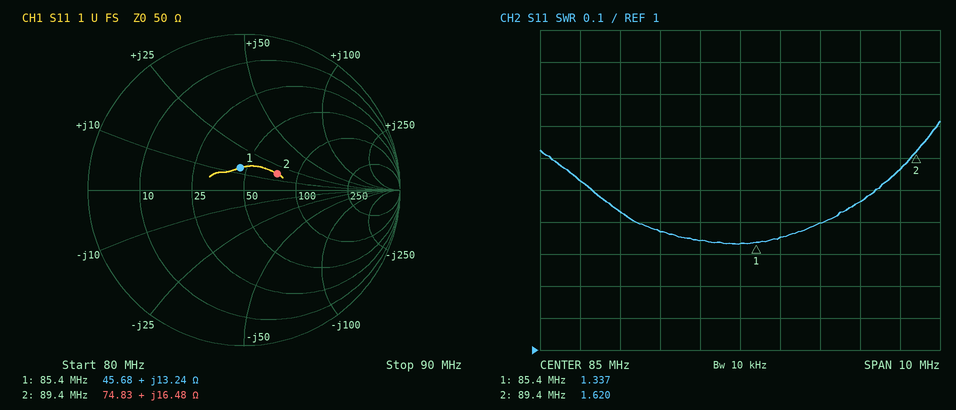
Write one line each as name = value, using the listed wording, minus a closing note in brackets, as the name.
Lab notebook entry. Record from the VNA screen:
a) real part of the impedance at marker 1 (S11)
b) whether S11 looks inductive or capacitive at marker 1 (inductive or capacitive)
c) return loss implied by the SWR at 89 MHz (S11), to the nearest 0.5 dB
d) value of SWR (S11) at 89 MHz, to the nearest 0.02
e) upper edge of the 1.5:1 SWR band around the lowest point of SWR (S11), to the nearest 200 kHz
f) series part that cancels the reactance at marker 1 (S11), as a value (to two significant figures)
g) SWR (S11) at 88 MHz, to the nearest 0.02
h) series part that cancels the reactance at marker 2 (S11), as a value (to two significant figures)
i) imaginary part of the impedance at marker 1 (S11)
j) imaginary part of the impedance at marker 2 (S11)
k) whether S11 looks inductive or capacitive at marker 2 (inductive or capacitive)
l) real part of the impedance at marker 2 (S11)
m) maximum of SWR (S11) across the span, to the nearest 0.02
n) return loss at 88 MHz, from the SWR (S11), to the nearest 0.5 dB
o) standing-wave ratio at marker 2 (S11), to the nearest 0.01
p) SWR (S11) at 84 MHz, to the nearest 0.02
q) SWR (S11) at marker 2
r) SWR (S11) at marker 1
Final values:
real part of the impedance at marker 1 = 45.68 Ω
whether S11 looks inductive or capacitive at marker 1 = inductive
return loss implied by the SWR at 89 MHz (S11), to the nearest 0.5 dB = 13.0 dB
value of SWR (S11) at 89 MHz, to the nearest 0.02 = 1.56
upper edge of the 1.5:1 SWR band around the lowest point of SWR (S11), to the nearest 200 kHz = 88.4 MHz
series part that cancels the reactance at marker 1 (S11), as a value = 140 pF
SWR (S11) at 88 MHz, to the nearest 0.02 = 1.46
series part that cancels the reactance at marker 2 (S11), as a value = 110 pF
imaginary part of the impedance at marker 1 = +13.24 Ω
imaginary part of the impedance at marker 2 = +16.48 Ω
whether S11 looks inductive or capacitive at marker 2 = inductive
real part of the impedance at marker 2 = 74.83 Ω
maximum of SWR (S11) across the span, to the nearest 0.02 = 1.72
return loss at 88 MHz, from the SWR (S11), to the nearest 0.5 dB = 14.5 dB
standing-wave ratio at marker 2 (S11), to the nearest 0.01 = 1.62
SWR (S11) at 84 MHz, to the nearest 0.02 = 1.34
SWR (S11) at marker 2 = 1.620
SWR (S11) at marker 1 = 1.337
